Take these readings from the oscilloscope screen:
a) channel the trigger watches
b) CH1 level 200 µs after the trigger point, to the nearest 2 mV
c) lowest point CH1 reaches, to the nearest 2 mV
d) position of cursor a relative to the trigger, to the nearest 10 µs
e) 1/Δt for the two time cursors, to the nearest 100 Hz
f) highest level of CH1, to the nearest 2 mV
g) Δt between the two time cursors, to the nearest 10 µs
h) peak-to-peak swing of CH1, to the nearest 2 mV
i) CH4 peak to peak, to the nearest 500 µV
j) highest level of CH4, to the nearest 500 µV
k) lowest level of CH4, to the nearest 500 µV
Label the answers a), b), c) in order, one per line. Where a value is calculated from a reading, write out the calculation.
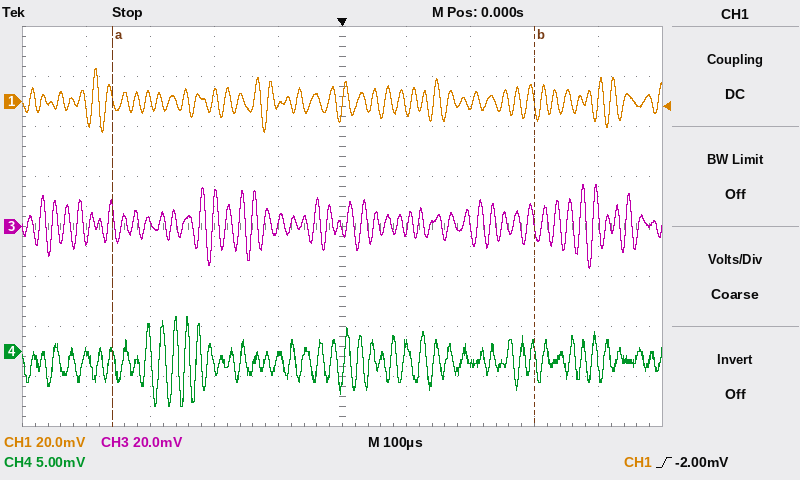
a) CH1
b) -2 mV
c) -12 mV
d) -360 µs
e) 1 / 660 µs ≈ 1.5 kHz
f) 14 mV
g) 660 µs
h) 14 mV − (-12 mV) = 26 mV
i) 3.5 mV − (-5.5 mV) = 9.0 mV
j) 3.5 mV
k) -5.5 mV
